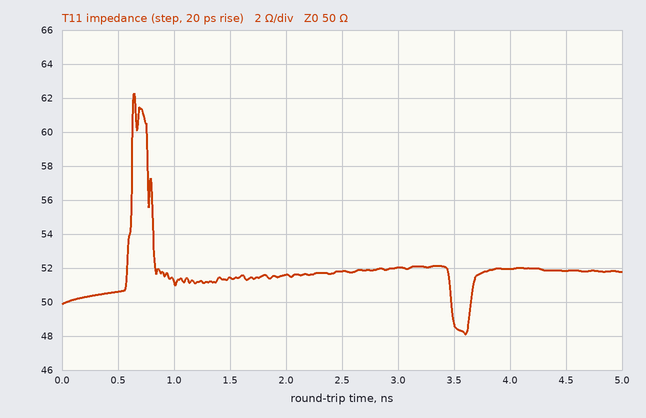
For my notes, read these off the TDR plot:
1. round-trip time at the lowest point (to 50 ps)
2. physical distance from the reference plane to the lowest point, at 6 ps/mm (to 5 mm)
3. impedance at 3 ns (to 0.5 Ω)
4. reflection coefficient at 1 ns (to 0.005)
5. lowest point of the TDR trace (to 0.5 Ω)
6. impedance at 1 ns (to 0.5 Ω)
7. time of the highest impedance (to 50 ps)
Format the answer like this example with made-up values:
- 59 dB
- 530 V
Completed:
- 3.60 ns
- 300 mm
- 52.0 Ω
- +0.010
- 48.0 Ω
- 51.0 Ω
- 650 ps
